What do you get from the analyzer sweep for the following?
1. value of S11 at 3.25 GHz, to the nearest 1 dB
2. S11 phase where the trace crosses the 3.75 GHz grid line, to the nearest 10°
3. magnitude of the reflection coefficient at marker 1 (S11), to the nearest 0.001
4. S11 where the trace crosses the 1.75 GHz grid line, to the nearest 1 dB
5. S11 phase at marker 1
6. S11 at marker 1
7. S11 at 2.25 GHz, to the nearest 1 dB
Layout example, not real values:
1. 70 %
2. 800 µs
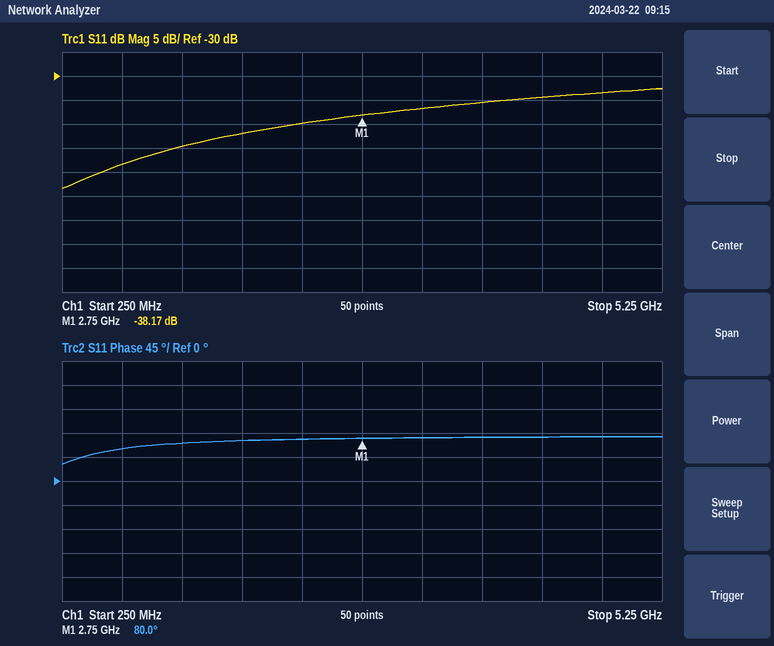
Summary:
1. -37 dB
2. 80°
3. 0.012
4. -42 dB
5. 80.0°
6. -38.17 dB
7. -40 dB
